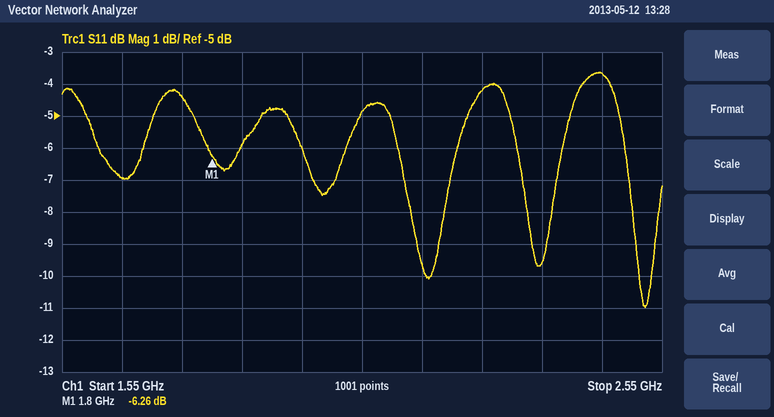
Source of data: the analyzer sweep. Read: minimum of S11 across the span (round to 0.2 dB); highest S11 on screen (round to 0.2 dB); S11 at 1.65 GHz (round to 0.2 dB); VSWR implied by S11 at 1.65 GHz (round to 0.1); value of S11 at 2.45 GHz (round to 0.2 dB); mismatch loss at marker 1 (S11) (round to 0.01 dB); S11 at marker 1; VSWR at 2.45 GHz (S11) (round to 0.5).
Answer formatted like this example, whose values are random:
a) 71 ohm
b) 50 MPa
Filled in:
a) -11.0 dB
b) -3.6 dB
c) -7.0 dB
d) 2.6
e) -3.6 dB
f) 1.17 dB
g) -6.26 dB
h) 5.0
